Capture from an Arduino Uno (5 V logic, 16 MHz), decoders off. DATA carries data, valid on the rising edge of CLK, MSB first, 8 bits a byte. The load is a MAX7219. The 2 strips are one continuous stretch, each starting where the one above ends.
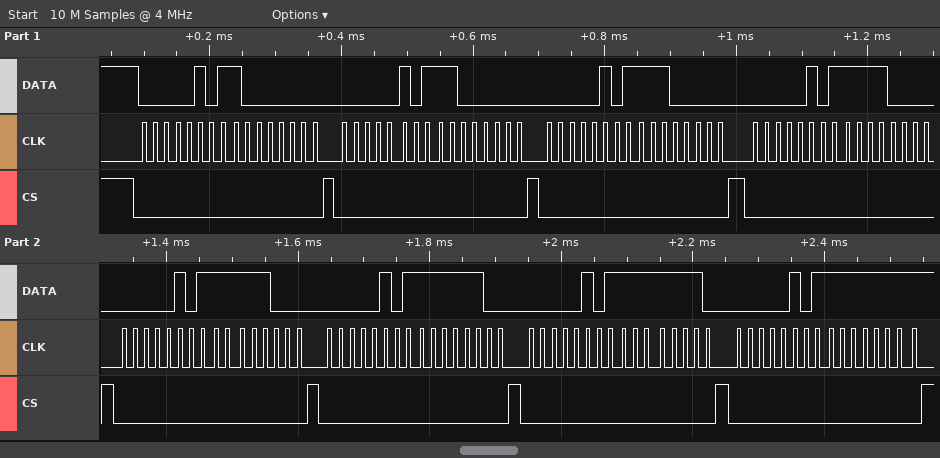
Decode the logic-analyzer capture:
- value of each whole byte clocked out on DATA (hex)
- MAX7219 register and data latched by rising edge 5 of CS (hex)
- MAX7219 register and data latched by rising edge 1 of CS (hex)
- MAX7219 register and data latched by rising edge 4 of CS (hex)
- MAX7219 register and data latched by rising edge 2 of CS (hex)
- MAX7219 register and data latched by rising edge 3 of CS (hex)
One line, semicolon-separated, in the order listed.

05 80 05 C0 05 E0 05 F0 05 F8 05 FC 05 FE 05 FF; register 0x5, data 0xF8; register 0x5, data 0x80; register 0x5, data 0xF0; register 0x5, data 0xC0; register 0x5, data 0xE0
